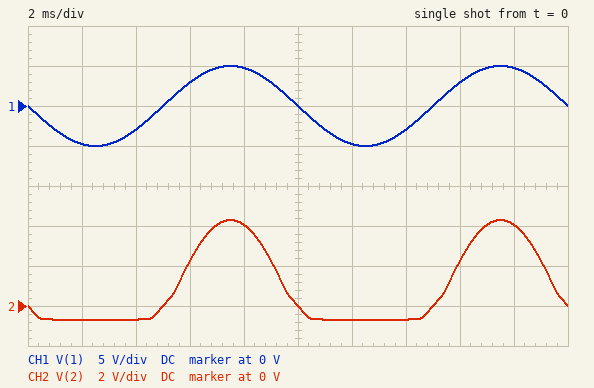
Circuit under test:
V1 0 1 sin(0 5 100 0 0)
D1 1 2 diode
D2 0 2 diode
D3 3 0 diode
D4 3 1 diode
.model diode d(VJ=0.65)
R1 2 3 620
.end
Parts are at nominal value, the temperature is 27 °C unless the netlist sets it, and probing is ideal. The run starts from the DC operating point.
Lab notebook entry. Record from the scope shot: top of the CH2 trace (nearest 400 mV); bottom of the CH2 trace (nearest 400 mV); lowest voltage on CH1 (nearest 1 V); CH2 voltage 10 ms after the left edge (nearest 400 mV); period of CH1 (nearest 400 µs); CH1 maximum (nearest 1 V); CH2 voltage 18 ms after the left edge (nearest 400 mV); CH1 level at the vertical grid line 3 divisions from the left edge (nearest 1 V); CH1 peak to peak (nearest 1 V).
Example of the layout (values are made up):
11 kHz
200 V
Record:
4.4 V
-800 mV
-5 V
0 V
10.0 ms
5 V
4.0 V
3 V
10 V
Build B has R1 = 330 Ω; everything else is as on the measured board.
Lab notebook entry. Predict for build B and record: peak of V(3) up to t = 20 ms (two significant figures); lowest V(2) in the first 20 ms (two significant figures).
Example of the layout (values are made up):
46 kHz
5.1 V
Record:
720 mV
-720 mV
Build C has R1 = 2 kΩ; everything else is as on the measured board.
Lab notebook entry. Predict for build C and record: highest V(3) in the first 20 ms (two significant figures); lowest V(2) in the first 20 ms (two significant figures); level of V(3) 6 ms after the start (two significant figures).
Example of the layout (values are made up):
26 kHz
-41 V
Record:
670 mV
-670 mV
650 mV
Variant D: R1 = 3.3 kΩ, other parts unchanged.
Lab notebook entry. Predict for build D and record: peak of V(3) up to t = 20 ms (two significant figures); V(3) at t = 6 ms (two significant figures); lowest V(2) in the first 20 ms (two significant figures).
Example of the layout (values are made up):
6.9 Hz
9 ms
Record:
660 mV
640 mV
-660 mV
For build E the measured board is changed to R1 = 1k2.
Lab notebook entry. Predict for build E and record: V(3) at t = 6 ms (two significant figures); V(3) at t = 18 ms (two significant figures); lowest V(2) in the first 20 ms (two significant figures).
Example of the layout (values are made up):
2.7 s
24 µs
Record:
660 mV
680 mV
-680 mV
